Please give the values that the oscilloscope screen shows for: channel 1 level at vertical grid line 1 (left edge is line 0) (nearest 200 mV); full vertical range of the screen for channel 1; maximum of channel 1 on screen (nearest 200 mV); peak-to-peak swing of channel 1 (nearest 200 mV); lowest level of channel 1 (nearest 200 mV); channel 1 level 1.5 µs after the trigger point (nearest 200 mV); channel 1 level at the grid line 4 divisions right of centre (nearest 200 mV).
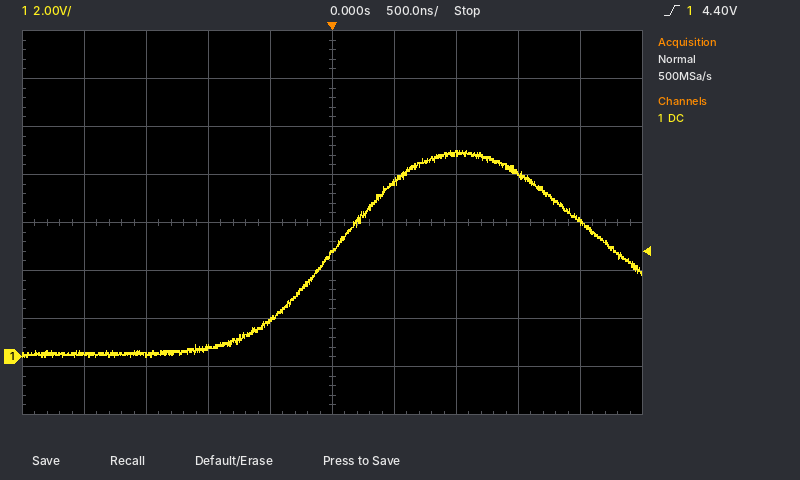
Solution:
200 mV
16 V
8.6 V
8.6 V
0.0 V
7.6 V
5.6 V
